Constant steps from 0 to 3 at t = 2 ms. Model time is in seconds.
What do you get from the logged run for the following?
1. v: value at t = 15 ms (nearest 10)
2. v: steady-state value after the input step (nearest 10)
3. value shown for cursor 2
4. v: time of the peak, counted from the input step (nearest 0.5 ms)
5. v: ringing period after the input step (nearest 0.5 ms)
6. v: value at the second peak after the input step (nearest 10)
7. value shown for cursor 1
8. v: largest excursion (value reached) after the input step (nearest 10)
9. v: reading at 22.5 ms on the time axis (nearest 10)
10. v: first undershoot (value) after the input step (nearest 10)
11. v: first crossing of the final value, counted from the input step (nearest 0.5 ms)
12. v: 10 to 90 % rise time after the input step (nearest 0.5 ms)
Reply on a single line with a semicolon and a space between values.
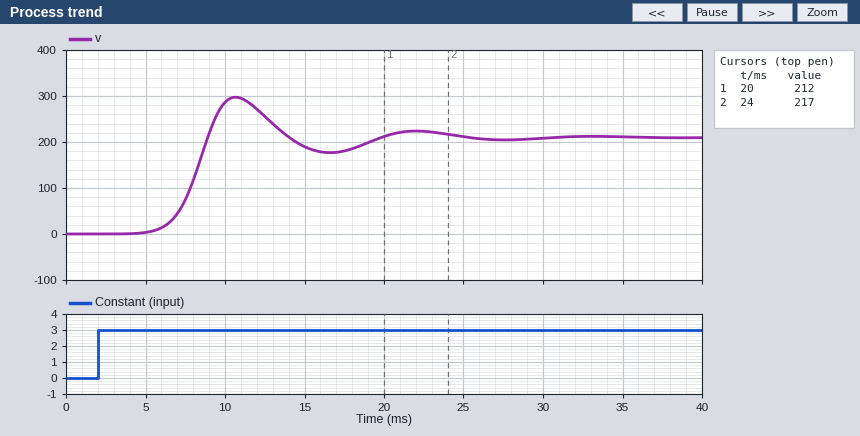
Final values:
190; 210; 217; 8.5 ms; 11.5 ms; 220; 212; 300; 220; 180; 7.0 ms; 2.5 ms
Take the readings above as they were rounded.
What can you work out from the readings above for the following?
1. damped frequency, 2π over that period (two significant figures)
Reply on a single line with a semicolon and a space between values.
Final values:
0.55 rad/ms
